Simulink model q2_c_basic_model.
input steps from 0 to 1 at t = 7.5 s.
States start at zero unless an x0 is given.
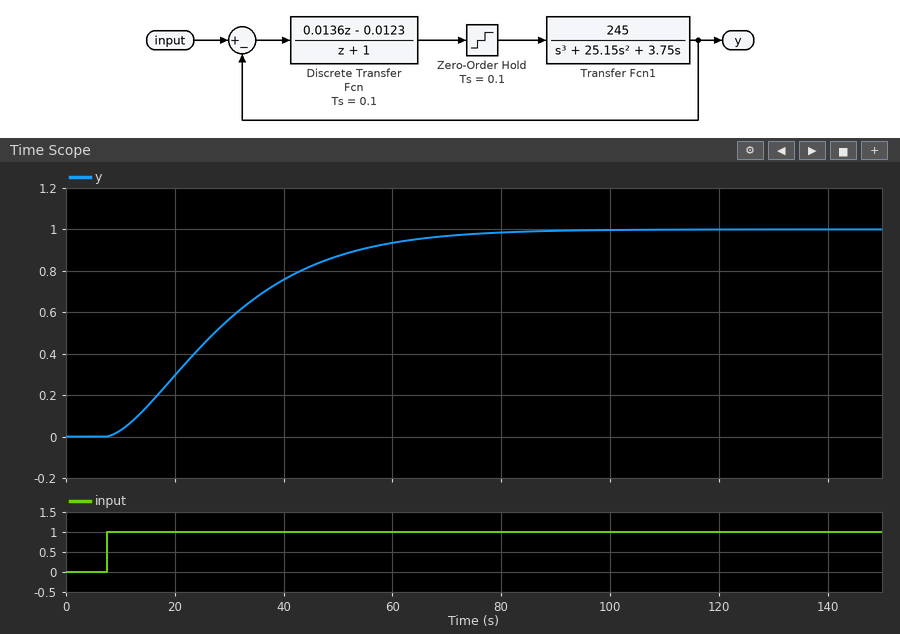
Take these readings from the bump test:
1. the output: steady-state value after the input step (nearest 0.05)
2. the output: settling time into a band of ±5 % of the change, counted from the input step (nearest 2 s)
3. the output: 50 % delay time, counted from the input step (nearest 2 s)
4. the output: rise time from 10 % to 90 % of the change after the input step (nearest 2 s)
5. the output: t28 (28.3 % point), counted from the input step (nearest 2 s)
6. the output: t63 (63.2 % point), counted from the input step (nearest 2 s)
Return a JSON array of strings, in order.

["1.00", "56 s", "20 s", "40 s", "12 s", "26 s"]
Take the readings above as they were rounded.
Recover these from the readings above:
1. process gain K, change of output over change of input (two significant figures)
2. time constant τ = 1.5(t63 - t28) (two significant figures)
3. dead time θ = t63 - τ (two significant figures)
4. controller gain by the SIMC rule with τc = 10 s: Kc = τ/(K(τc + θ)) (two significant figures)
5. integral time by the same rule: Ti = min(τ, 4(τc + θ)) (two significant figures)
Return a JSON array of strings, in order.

["1.0", "21 s", "5.0 s", "1.4", "21 s"]
